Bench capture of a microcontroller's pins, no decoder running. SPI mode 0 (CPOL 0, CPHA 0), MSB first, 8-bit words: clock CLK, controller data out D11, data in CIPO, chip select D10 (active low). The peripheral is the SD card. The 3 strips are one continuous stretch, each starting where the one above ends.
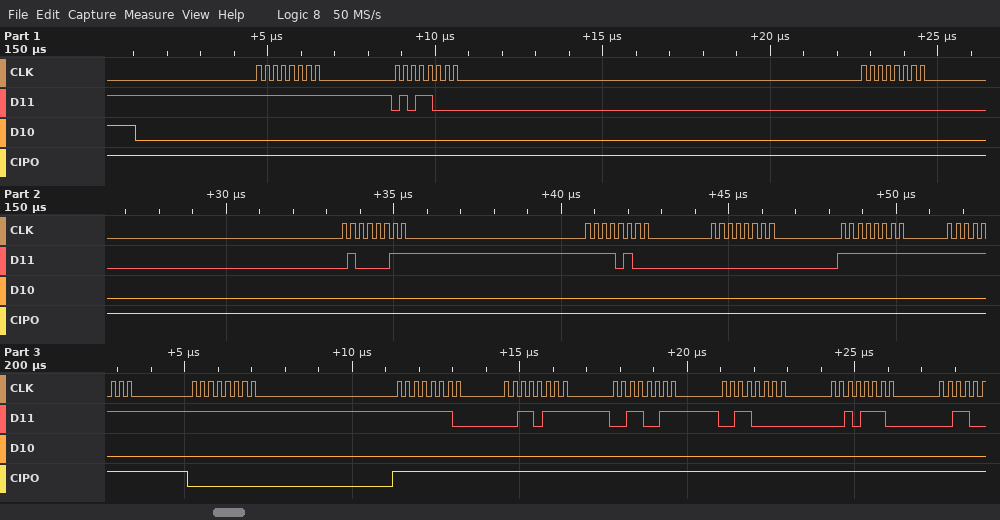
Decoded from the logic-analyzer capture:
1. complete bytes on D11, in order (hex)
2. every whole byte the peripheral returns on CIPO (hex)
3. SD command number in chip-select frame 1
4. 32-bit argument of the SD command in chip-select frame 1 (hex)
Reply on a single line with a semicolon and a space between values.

FF 58 00 43 F4 00 FF FF FF FE 37 33 30 2E; FF FF FF FF FF FF FF FF 00 FF FF FF FF FF; CMD24; 0x0043F400
